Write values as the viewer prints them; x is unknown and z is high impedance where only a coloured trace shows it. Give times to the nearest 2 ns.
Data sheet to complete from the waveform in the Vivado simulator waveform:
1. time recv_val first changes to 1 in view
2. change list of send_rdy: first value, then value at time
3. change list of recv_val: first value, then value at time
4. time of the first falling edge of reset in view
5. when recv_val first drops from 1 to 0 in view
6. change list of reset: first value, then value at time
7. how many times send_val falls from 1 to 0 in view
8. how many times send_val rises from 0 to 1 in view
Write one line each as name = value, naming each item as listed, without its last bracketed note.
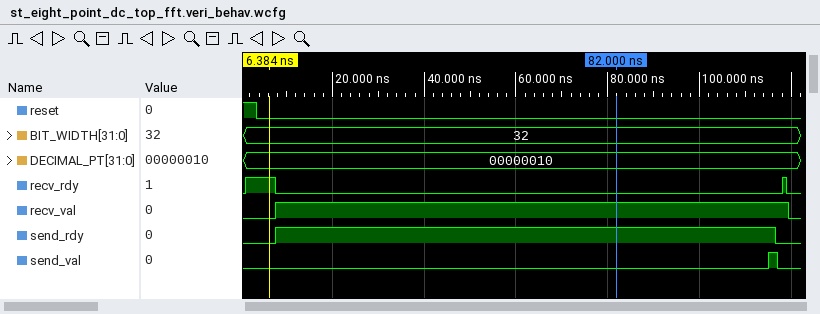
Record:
time recv_val first changes to 1 in view = 8 ns
change list of send_rdy: first value, then value at time = 0, 1 at 8 ns, 0 at 116 ns
change list of recv_val: first value, then value at time = 0, 1 at 8 ns, 0 at 120 ns
time of the first falling edge of reset in view = 4 ns
when recv_val first drops from 1 to 0 in view = 120 ns
change list of reset: first value, then value at time = 1, 0 at 4 ns
how many times send_val falls from 1 to 0 in view = 1
how many times send_val rises from 0 to 1 in view = 1
